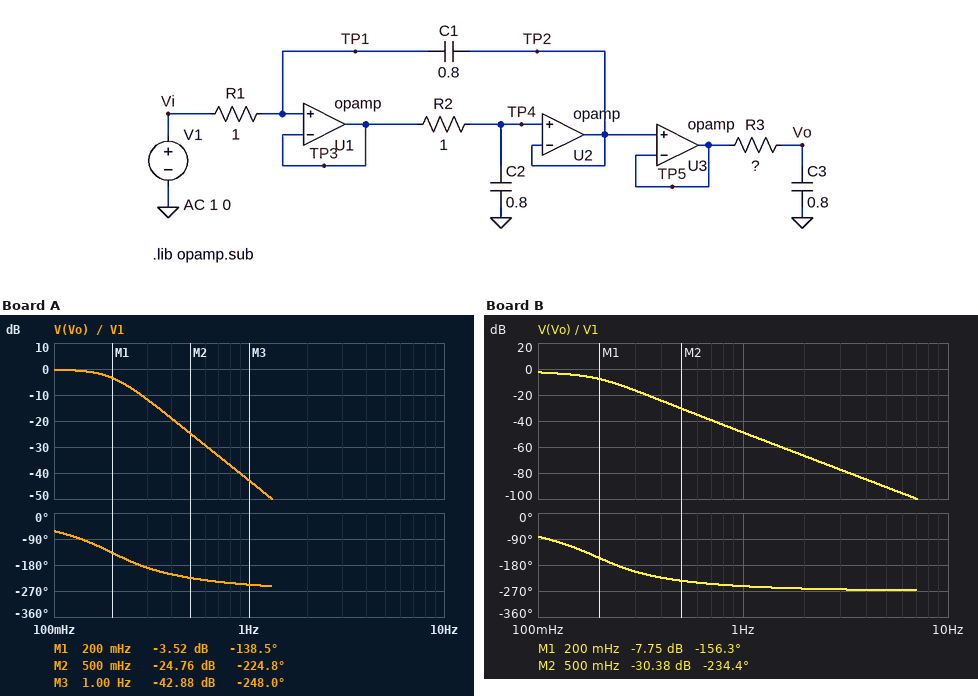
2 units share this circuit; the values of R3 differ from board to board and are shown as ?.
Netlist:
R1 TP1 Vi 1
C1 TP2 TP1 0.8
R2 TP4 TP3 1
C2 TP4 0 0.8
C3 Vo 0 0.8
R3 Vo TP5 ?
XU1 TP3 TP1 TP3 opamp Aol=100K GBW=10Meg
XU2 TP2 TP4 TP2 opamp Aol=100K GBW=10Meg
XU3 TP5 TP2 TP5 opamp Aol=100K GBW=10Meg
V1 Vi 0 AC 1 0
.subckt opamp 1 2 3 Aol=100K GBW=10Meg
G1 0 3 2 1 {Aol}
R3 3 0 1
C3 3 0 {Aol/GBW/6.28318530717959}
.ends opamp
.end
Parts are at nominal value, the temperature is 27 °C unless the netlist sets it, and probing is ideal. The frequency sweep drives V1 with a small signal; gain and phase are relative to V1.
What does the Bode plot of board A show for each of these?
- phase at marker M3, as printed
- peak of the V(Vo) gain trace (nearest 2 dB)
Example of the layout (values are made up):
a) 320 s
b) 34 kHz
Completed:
a) -248.0 deg
b) 0 dB
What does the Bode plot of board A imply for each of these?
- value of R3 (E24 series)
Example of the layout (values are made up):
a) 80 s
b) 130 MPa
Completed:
a) 1.1 Ω
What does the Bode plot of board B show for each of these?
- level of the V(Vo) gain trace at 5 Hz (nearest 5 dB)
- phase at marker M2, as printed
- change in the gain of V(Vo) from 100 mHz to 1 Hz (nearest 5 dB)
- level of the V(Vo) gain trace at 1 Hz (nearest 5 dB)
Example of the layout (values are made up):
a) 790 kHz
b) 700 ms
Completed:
a) -90 dB
b) -234.4 deg
c) -45 dB
d) -50 dB
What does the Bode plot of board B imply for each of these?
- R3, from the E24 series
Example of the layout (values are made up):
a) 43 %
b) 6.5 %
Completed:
a) 2.2 Ω
